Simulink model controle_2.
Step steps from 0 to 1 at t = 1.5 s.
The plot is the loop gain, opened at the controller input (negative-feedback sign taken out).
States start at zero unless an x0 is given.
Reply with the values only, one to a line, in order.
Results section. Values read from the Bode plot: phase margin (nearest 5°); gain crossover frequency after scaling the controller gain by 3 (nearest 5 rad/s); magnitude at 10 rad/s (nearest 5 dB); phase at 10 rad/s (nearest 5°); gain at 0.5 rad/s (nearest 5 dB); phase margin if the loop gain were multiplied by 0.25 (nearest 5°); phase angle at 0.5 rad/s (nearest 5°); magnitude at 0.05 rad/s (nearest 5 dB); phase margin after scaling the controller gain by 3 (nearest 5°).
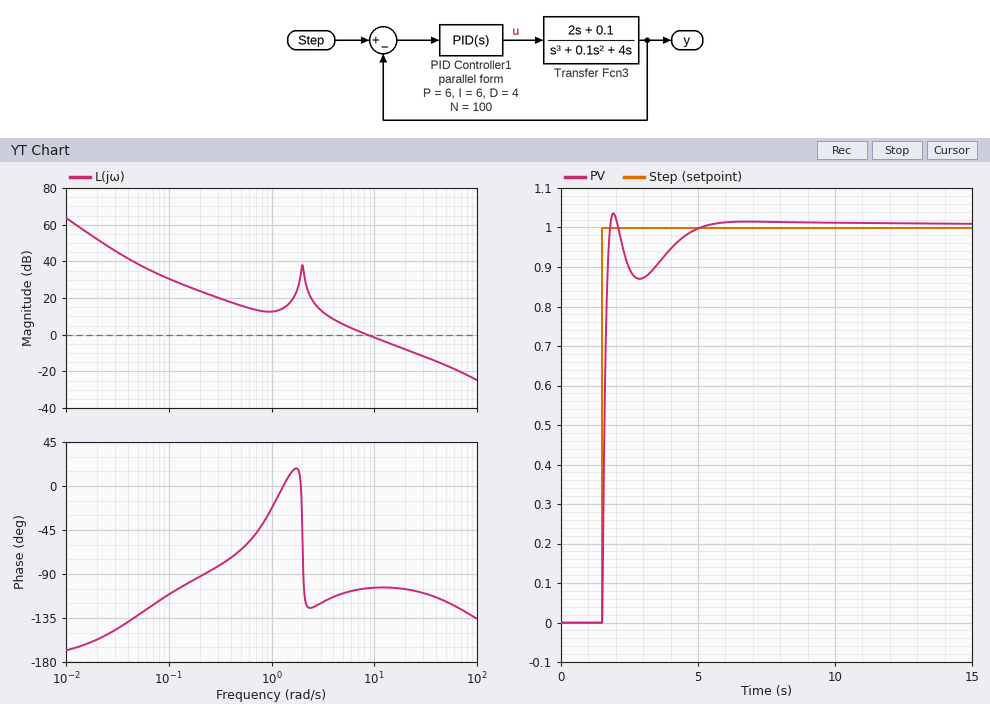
75°
25 rad/s
0 dB
-105°
15 dB
60°
-65°
40 dB
75°
